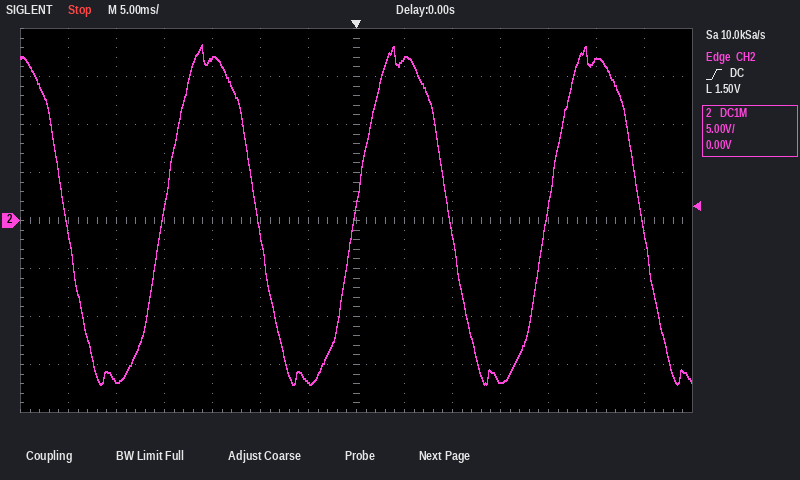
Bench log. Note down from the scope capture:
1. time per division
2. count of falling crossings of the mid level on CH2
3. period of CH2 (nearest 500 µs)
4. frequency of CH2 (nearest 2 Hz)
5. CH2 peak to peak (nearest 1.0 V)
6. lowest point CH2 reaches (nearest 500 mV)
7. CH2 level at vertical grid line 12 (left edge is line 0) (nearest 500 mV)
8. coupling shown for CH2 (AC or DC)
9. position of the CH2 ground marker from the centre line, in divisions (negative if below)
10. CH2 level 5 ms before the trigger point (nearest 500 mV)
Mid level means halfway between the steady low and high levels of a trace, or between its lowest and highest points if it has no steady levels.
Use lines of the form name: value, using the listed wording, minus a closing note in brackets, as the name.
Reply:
time per division: 5 ms
count of falling crossings of the mid level on CH2: 4
period of CH2: 20.0 ms
frequency of CH2: 50 Hz
CH2 peak to peak: 35.0 V
lowest point CH2 reaches: -17.0 V
CH2 level at vertical grid line 12 (left edge is line 0): 16.5 V
coupling shown for CH2: DC
position of the CH2 ground marker from the centre line, in divisions: 0.0 div
CH2 level 5 ms before the trigger point: -17.0 V
